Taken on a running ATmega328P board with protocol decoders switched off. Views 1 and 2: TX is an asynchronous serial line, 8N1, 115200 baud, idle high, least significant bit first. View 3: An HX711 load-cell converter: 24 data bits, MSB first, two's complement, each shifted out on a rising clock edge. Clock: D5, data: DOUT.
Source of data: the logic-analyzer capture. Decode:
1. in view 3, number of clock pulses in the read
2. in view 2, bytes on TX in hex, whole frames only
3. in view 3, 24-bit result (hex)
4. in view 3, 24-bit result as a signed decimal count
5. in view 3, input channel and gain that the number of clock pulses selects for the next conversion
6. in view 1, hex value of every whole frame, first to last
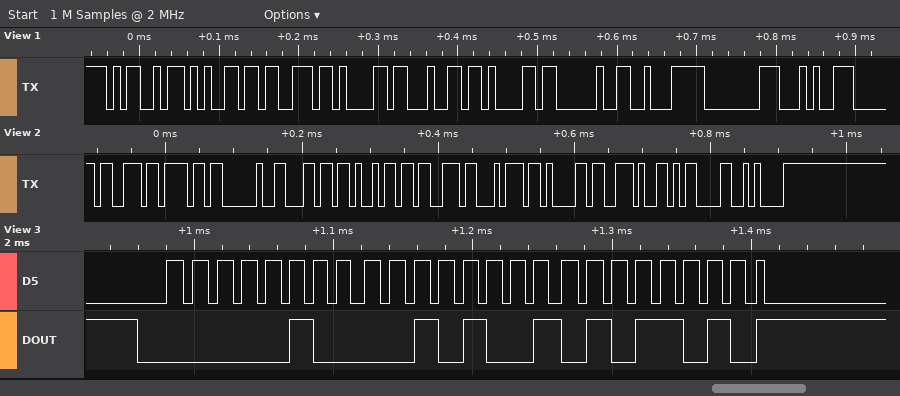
25
0x73 0x6F 0x20 0x6C 0x69 0x73 0x74 0x61 0x2E 0x0D 0x0A
0x04295A
272730
channel A, gain 128
4D 65 73 61 64 61 20 E2 80 94
